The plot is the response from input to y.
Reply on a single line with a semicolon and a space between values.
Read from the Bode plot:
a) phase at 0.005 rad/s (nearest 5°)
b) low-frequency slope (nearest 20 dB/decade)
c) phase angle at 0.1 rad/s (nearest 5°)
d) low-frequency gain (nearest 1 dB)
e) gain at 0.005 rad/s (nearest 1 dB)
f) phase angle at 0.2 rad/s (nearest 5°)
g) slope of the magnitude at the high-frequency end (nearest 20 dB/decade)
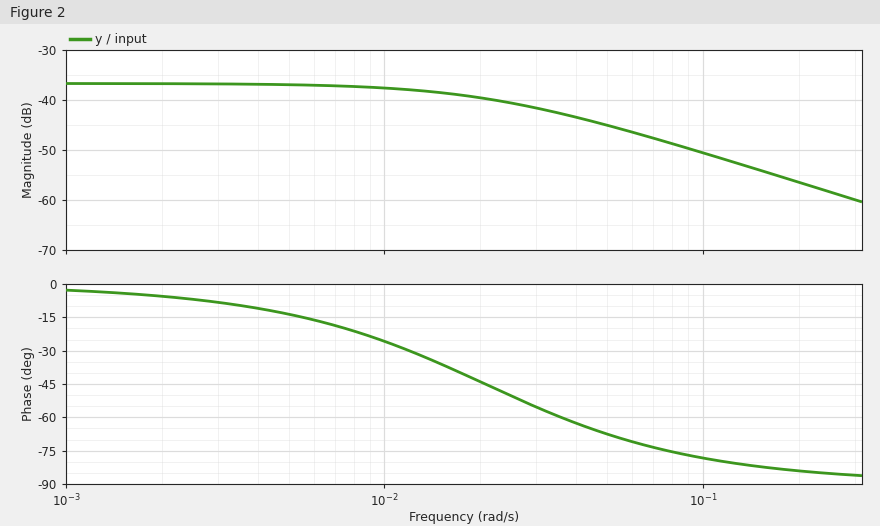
-15°; 0 dB/decade; -80°; -37 dB; -37 dB; -85°; -20 dB/decade
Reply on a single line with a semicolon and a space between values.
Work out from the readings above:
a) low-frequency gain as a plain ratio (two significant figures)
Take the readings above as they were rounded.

0.014
